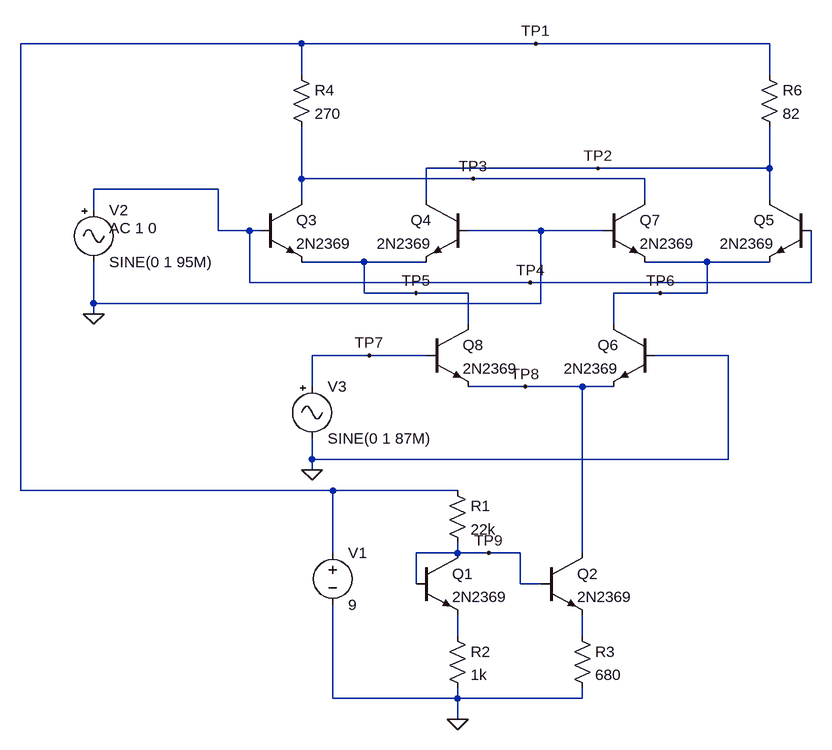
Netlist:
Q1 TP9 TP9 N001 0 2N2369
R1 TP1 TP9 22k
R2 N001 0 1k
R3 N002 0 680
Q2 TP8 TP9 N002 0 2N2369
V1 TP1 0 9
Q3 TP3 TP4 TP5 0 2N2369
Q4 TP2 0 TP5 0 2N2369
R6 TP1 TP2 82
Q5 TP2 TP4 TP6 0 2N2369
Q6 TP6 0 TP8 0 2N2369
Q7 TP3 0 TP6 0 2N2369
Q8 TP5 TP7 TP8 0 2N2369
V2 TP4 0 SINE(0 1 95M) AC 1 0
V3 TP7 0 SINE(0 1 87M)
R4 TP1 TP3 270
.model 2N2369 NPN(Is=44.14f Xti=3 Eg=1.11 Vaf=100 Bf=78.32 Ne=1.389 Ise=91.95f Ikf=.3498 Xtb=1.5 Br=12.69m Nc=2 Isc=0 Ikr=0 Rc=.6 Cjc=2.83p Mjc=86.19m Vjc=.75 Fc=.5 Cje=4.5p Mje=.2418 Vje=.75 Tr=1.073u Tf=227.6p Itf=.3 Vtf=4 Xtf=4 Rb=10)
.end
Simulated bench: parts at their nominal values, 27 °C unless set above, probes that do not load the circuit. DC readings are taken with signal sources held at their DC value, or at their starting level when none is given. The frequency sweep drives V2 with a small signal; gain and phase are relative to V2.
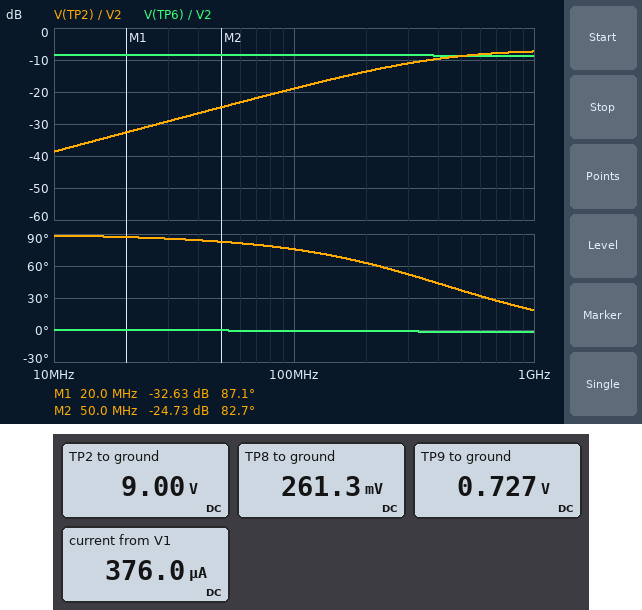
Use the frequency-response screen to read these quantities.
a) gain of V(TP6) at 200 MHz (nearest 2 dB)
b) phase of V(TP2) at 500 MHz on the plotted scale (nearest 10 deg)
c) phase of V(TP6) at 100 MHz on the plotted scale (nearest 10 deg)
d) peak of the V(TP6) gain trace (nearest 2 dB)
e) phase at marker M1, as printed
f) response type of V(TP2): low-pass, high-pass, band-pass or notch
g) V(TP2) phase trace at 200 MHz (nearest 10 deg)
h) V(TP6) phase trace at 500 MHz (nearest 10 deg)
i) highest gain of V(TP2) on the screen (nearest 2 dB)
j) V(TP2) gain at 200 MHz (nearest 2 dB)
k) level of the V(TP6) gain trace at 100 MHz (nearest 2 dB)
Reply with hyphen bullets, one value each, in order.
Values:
- -8 dB
- 40 deg
- 0 deg
- -8 dB
- 87.1 deg
- high-pass
- 60 deg
- 0 deg
- -8 dB
- -14 dB
- -8 dB
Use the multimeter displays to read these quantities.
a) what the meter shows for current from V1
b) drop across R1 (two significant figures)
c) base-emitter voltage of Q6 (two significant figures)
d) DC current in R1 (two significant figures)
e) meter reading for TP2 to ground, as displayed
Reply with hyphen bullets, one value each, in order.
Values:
- 376.0 µA
- 8.3 V
- -260 mV
- 380 µA
- 9.00 V
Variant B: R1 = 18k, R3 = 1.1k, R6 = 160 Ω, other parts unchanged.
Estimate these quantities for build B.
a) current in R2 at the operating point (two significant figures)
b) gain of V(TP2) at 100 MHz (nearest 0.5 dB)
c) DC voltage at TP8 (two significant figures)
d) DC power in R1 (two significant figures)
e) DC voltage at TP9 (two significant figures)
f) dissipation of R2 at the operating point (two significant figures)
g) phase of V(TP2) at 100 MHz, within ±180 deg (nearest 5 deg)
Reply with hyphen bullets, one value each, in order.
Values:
- 240 µA
- -13.5 dB
- 350 mV
- 3.7 mW
- 820 mV
- 57 µW
- 65 deg
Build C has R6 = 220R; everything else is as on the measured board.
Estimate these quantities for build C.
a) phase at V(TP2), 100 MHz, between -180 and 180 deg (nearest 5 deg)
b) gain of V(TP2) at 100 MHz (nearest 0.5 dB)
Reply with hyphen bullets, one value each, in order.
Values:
- 55 deg
- -11.5 dB
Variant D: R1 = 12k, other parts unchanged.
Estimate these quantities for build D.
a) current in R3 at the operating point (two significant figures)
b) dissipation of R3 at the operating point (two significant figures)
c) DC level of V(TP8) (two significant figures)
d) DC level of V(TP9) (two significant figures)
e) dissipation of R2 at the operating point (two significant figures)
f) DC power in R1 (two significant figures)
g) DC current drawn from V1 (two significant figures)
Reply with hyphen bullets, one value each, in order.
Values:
- 400 µA
- 110 µW
- 380 mV
- 870 mV
- 80 µW
- 5.5 mW
- 680 µA
